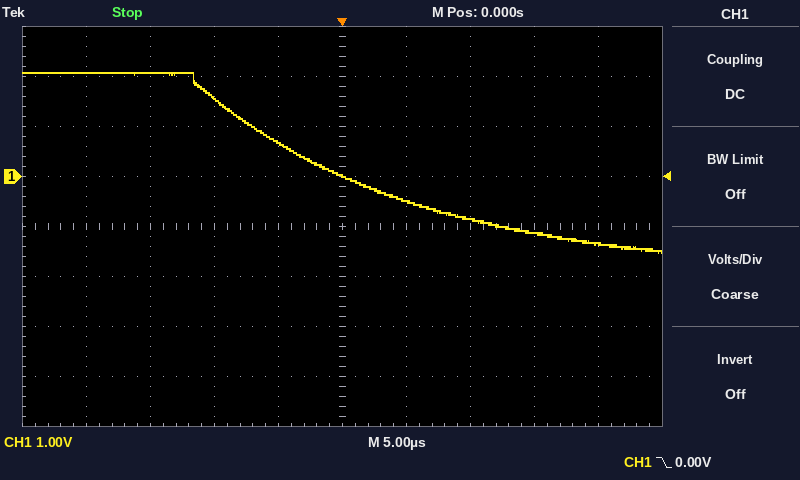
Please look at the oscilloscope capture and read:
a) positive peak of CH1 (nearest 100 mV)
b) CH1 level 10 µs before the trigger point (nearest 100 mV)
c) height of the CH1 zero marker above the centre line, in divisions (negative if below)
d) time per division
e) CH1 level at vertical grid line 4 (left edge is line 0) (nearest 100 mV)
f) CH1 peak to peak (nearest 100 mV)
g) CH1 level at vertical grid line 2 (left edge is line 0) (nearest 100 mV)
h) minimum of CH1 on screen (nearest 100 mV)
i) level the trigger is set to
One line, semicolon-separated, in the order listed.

2.1 V; 1.6 V; +1.0 div; 5 µs; 700 mV; 3.6 V; 2.1 V; -1.5 V; 0.00 V
